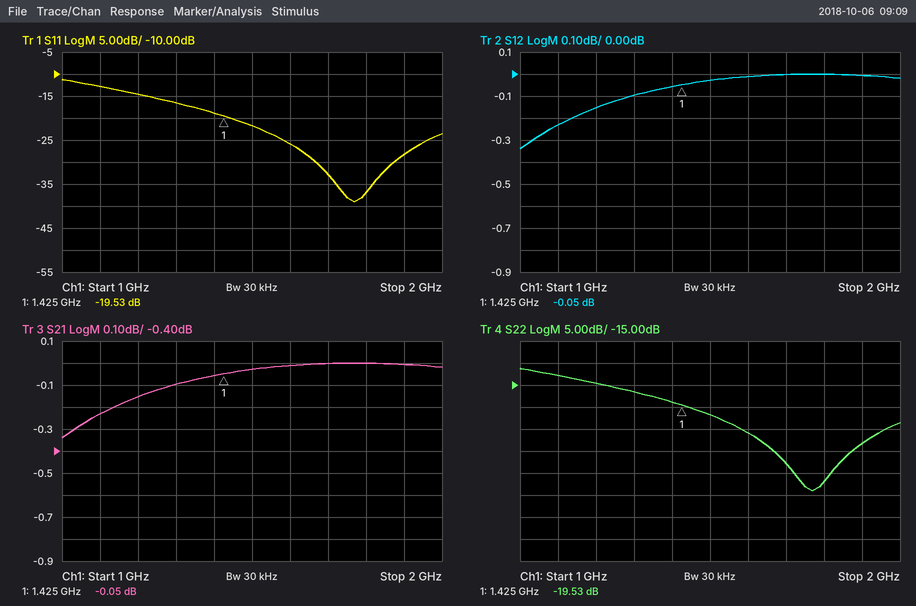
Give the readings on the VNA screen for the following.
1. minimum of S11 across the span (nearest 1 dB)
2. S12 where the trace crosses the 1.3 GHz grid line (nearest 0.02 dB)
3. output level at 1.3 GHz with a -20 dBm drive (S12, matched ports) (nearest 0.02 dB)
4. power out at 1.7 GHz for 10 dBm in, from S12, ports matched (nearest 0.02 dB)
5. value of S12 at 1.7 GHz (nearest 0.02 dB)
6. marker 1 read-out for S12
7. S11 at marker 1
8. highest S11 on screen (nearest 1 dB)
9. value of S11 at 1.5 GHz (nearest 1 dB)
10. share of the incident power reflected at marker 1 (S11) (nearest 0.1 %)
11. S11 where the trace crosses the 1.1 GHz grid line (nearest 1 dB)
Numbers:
-39 dB
-0.10 dB
-20.10 dBm
10.00 dBm
0.00 dB
-0.05 dB
-19.53 dB
-11 dB
-22 dB
1.1 %
-13 dB
